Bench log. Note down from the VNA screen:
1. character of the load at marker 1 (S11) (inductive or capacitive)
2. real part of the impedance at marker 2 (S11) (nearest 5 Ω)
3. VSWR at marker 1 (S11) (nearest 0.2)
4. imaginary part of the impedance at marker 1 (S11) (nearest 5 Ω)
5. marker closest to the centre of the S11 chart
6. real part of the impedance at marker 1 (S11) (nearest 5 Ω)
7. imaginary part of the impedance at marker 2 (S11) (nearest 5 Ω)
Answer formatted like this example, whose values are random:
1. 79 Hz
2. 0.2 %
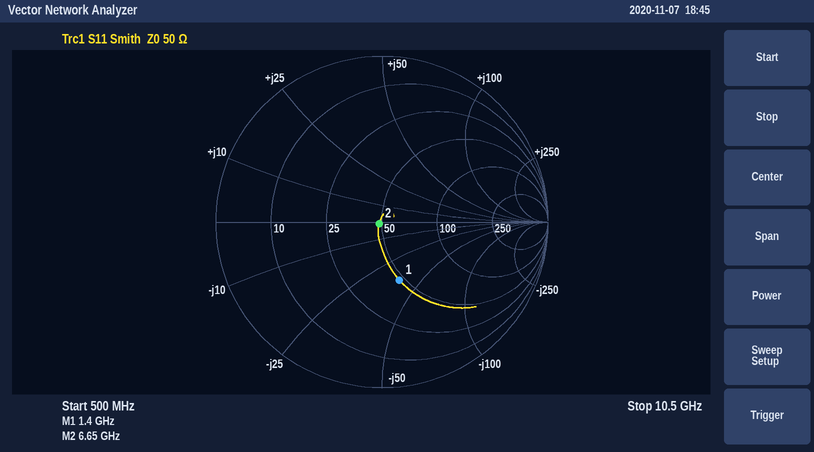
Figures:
1. capacitive
2. 50 Ω
3. 2.2
4. -40 Ω
5. marker 2
6. 45 Ω
7. 0 Ω
